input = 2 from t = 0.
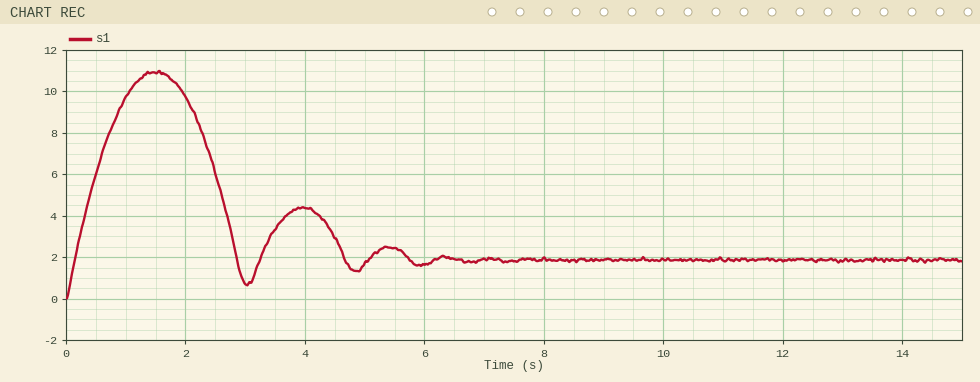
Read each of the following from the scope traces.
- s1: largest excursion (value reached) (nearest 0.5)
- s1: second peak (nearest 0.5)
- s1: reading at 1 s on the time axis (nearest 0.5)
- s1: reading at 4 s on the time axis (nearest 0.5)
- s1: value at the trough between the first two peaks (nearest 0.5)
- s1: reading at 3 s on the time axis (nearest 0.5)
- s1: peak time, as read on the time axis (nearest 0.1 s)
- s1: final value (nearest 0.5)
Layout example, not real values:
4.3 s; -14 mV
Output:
11.0; 4.5; 9.5; 4.5; 0.5; 0.5; 1.5 s; 2.0
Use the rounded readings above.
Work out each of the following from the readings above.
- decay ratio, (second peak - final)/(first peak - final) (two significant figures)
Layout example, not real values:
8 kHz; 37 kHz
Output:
0.28
